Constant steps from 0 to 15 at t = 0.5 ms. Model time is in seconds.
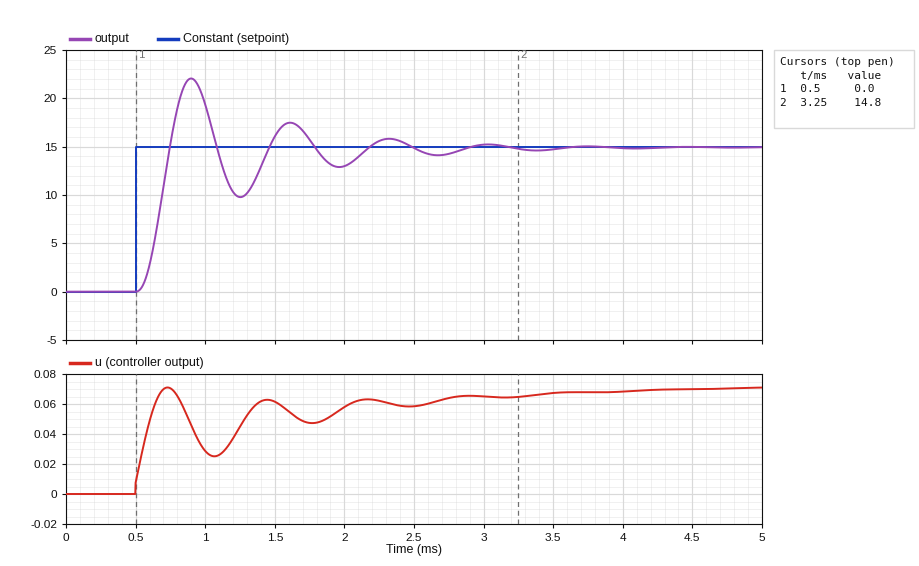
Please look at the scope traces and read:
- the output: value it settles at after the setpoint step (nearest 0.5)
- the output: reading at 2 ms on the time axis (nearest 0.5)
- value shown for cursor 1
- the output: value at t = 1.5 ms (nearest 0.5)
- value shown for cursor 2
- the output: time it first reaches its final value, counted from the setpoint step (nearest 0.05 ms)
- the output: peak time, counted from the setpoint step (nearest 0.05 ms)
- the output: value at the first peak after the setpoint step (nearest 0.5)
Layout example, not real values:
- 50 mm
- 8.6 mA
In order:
- 15.0
- 13.0
- 0.0
- 16.0
- 14.8
- 0.25 ms
- 0.40 ms
- 22.0
